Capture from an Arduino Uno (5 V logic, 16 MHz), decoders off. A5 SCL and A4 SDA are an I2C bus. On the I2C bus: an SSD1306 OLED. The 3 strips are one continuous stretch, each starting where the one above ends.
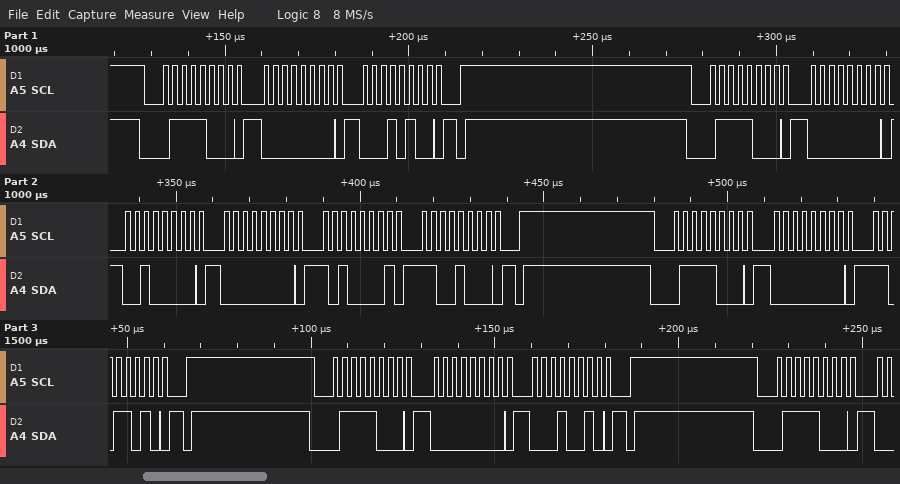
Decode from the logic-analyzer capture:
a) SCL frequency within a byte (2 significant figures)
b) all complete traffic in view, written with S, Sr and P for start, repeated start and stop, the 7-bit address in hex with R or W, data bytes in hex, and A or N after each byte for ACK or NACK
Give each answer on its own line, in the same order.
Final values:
400 kHz
S 3CW A 00 A 14 A P S 3CW A 00 A 20 A 00 A A1 A C8 A P S 3CW A 00 A DA A P S 3CW A 00 A 12 A P S 3CW A
